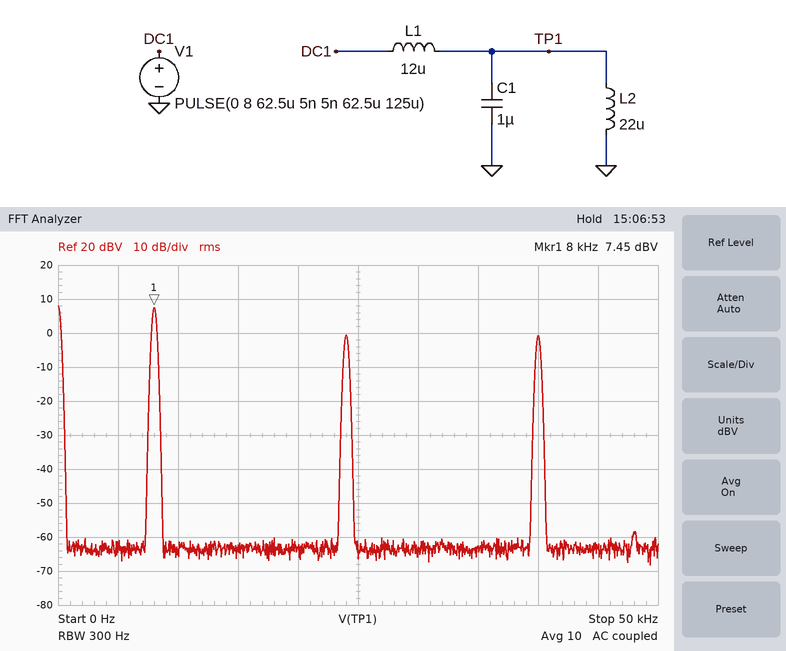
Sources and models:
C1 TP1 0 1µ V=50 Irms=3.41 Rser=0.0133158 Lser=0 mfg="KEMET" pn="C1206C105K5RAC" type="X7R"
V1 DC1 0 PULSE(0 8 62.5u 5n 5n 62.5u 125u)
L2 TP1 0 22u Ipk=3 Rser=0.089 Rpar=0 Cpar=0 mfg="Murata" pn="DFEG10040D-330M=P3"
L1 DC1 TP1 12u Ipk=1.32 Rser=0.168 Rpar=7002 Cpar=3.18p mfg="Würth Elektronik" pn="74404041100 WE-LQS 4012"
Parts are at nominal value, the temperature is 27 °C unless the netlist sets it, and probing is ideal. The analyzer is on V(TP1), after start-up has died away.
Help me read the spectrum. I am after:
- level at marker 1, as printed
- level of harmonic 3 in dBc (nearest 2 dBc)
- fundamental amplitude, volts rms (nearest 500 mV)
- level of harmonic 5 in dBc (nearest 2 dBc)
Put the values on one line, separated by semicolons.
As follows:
7.45 dBV; -8 dBc; 2.5 V; -8 dBc
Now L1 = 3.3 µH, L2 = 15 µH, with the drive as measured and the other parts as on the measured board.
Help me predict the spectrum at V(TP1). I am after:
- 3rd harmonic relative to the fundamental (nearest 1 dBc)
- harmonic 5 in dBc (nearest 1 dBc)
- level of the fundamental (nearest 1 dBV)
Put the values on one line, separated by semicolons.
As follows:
-9 dBc; -12 dBc; 9 dBV
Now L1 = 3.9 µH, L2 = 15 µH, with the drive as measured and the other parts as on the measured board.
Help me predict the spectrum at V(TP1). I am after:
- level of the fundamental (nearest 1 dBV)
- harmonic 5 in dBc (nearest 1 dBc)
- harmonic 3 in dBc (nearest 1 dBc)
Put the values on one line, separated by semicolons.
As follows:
9 dBV; -12 dBc; -9 dBc
